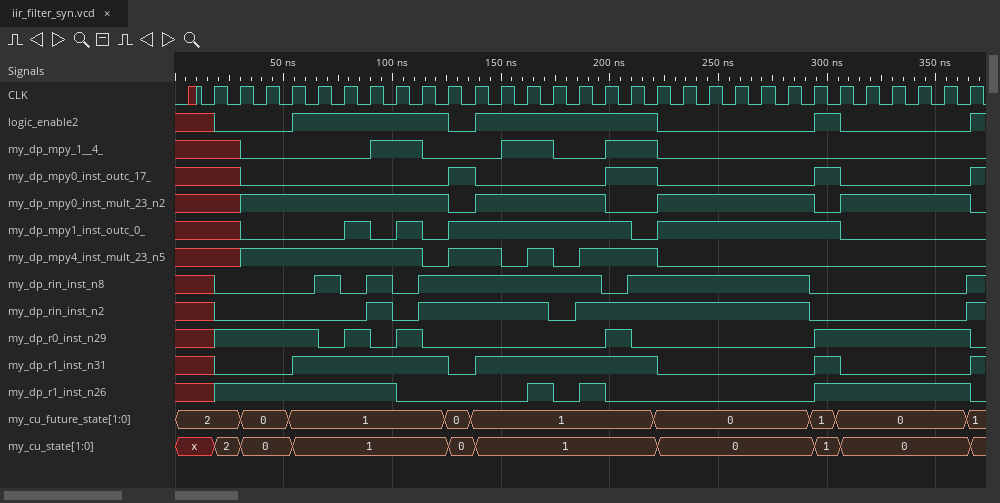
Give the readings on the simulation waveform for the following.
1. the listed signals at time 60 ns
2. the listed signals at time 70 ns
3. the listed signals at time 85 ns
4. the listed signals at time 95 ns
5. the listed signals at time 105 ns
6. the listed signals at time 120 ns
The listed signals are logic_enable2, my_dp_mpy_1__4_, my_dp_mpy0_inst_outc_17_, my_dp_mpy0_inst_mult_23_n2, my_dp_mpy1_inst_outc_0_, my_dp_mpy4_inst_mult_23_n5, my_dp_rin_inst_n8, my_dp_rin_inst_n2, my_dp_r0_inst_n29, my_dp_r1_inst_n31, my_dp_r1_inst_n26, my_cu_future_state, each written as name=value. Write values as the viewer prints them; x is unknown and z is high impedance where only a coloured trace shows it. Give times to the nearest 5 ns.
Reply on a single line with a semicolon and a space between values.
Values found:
logic_enable2=1, my_dp_mpy_1__4_=0, my_dp_mpy0_inst_outc_17_=0, my_dp_mpy0_inst_mult_23_n2=1, my_dp_mpy1_inst_outc_0_=0, my_dp_mpy4_inst_mult_23_n5=1, my_dp_rin_inst_n8=0, my_dp_rin_inst_n2=0, my_dp_r0_inst_n29=1, my_dp_r1_inst_n31=1, my_dp_r1_inst_n26=1, my_cu_future_state=1; logic_enable2=1, my_dp_mpy_1__4_=0, my_dp_mpy0_inst_outc_17_=0, my_dp_mpy0_inst_mult_23_n2=1, my_dp_mpy1_inst_outc_0_=0, my_dp_mpy4_inst_mult_23_n5=1, my_dp_rin_inst_n8=1, my_dp_rin_inst_n2=0, my_dp_r0_inst_n29=0, my_dp_r1_inst_n31=1, my_dp_r1_inst_n26=1, my_cu_future_state=1; logic_enable2=1, my_dp_mpy_1__4_=0, my_dp_mpy0_inst_outc_17_=0, my_dp_mpy0_inst_mult_23_n2=1, my_dp_mpy1_inst_outc_0_=1, my_dp_mpy4_inst_mult_23_n5=1, my_dp_rin_inst_n8=0, my_dp_rin_inst_n2=0, my_dp_r0_inst_n29=1, my_dp_r1_inst_n31=1, my_dp_r1_inst_n26=1, my_cu_future_state=1; logic_enable2=1, my_dp_mpy_1__4_=1, my_dp_mpy0_inst_outc_17_=0, my_dp_mpy0_inst_mult_23_n2=1, my_dp_mpy1_inst_outc_0_=0, my_dp_mpy4_inst_mult_23_n5=1, my_dp_rin_inst_n8=1, my_dp_rin_inst_n2=1, my_dp_r0_inst_n29=0, my_dp_r1_inst_n31=1, my_dp_r1_inst_n26=1, my_cu_future_state=1; logic_enable2=1, my_dp_mpy_1__4_=1, my_dp_mpy0_inst_outc_17_=0, my_dp_mpy0_inst_mult_23_n2=1, my_dp_mpy1_inst_outc_0_=1, my_dp_mpy4_inst_mult_23_n5=1, my_dp_rin_inst_n8=0, my_dp_rin_inst_n2=0, my_dp_r0_inst_n29=1, my_dp_r1_inst_n31=1, my_dp_r1_inst_n26=0, my_cu_future_state=1; logic_enable2=1, my_dp_mpy_1__4_=0, my_dp_mpy0_inst_outc_17_=0, my_dp_mpy0_inst_mult_23_n2=1, my_dp_mpy1_inst_outc_0_=0, my_dp_mpy4_inst_mult_23_n5=0, my_dp_rin_inst_n8=1, my_dp_rin_inst_n2=1, my_dp_r0_inst_n29=0, my_dp_r1_inst_n31=1, my_dp_r1_inst_n26=0, my_cu_future_state=1
